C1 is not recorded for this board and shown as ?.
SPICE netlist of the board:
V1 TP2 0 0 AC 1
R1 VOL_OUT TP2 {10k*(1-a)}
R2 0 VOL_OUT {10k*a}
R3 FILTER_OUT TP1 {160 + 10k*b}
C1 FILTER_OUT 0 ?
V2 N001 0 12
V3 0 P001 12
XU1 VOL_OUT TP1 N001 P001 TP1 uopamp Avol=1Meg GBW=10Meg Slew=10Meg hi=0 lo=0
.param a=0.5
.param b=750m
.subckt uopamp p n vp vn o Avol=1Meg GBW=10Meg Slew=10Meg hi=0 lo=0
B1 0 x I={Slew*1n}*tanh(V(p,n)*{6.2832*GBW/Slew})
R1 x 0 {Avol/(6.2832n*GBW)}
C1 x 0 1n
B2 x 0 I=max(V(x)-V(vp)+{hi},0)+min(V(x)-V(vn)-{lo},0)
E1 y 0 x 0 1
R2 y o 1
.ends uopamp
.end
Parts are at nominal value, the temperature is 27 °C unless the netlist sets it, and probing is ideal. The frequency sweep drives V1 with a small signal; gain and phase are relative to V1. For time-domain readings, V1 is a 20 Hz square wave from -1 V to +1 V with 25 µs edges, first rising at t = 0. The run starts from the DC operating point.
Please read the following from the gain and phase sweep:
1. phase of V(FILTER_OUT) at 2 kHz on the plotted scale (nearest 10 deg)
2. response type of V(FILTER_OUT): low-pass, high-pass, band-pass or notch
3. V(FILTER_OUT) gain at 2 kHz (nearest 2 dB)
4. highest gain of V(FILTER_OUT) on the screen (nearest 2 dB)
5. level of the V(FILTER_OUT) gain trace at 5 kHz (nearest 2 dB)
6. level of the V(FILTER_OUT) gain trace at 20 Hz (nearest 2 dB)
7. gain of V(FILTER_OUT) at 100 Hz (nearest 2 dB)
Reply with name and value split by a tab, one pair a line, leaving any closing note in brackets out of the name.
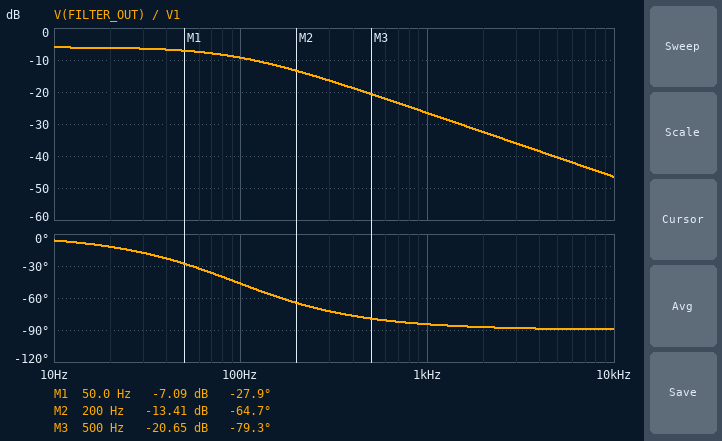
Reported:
phase of V(FILTER_OUT) at 2 kHz on the plotted scale	-90 deg
response type of V(FILTER_OUT): low-pass, high-pass, band-pass or notch	low-pass
V(FILTER_OUT) gain at 2 kHz	-32 dB
highest gain of V(FILTER_OUT) on the screen	-6 dB
level of the V(FILTER_OUT) gain trace at 5 kHz	-40 dB
level of the V(FILTER_OUT) gain trace at 20 Hz	-6 dB
gain of V(FILTER_OUT) at 100 Hz	-10 dB
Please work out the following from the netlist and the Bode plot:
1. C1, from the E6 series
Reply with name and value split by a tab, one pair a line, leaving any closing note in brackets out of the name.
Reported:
C1, from the E6 series	220 nF
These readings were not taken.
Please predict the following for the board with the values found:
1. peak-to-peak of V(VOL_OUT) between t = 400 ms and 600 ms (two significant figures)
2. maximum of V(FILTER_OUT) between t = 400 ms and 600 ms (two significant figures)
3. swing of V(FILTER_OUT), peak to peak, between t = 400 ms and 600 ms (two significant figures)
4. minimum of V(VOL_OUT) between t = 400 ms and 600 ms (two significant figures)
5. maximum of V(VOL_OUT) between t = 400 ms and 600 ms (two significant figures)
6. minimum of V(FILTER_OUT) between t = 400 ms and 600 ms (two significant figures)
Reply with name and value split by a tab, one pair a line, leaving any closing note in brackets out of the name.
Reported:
peak-to-peak of V(VOL_OUT) between t = 400 ms and 600 ms	1.0 V
maximum of V(FILTER_OUT) between t = 400 ms and 600 ms	500 mV
swing of V(FILTER_OUT), peak to peak, between t = 400 ms and 600 ms	1.0 V
minimum of V(VOL_OUT) between t = 400 ms and 600 ms	-500 mV
maximum of V(VOL_OUT) between t = 400 ms and 600 ms	500 mV
minimum of V(FILTER_OUT) between t = 400 ms and 600 ms	-500 mV
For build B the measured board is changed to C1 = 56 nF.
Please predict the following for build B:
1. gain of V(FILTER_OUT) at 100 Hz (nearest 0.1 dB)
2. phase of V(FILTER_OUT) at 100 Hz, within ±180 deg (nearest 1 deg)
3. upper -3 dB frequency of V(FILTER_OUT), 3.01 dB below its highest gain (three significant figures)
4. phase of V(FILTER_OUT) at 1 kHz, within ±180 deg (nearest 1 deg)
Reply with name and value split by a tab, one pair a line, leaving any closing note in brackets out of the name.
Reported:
gain of V(FILTER_OUT) at 100 Hz	-6.3 dB
phase of V(FILTER_OUT) at 100 Hz, within ±180 deg	-15 deg
upper -3 dB frequency of V(FILTER_OUT), 3.01 dB below its highest gain	371 Hz
phase of V(FILTER_OUT) at 1 kHz, within ±180 deg	-70 deg
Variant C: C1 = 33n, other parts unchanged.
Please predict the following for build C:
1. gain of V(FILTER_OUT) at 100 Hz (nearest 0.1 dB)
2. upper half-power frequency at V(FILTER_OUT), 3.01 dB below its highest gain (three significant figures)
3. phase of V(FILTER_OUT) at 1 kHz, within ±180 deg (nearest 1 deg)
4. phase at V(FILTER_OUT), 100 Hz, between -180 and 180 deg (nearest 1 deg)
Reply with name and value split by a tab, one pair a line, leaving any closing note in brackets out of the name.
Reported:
gain of V(FILTER_OUT) at 100 Hz	-6.1 dB
upper half-power frequency at V(FILTER_OUT), 3.01 dB below its highest gain	630 Hz
phase of V(FILTER_OUT) at 1 kHz, within ±180 deg	-58 deg
phase at V(FILTER_OUT), 100 Hz, between -180 and 180 deg	-9 deg
